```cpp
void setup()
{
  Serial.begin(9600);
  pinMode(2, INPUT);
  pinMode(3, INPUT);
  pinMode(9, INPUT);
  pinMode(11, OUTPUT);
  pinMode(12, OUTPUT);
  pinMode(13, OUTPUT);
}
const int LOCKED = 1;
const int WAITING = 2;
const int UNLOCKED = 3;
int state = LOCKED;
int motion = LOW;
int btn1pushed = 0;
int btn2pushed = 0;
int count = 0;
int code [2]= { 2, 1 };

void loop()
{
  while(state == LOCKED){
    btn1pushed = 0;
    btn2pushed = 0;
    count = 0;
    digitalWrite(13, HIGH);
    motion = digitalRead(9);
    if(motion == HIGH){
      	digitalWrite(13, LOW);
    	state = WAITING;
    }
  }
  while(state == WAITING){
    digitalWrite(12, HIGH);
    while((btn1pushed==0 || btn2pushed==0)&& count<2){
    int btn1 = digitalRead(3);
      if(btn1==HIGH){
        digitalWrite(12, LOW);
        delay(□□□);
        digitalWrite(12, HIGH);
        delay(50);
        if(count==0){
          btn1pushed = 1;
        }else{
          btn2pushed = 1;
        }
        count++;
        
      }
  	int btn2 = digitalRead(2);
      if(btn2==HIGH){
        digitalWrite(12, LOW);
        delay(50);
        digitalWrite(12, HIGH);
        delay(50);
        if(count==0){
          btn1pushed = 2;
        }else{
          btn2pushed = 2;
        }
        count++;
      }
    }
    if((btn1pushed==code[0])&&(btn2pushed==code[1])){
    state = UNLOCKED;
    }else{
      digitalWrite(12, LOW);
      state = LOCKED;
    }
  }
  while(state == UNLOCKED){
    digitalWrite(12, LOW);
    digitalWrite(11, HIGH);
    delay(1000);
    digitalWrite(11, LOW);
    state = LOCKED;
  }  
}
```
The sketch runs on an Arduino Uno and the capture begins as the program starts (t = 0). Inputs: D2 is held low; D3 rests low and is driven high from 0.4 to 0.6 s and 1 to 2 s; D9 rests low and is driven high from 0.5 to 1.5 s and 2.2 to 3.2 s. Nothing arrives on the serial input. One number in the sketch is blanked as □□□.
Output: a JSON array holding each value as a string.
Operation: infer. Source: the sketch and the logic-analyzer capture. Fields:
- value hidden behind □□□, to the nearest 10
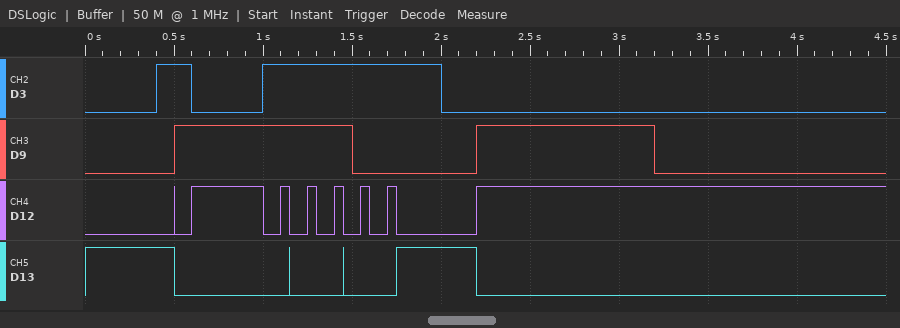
["100"]
